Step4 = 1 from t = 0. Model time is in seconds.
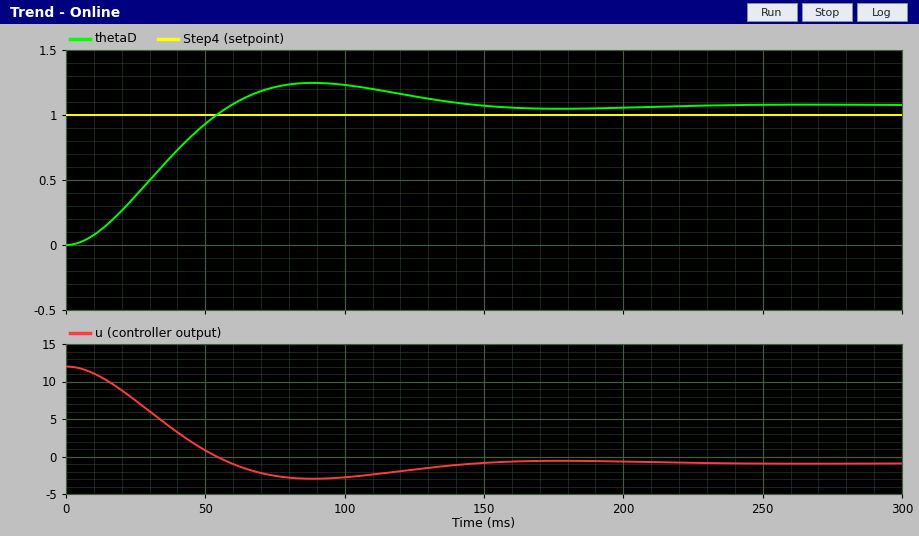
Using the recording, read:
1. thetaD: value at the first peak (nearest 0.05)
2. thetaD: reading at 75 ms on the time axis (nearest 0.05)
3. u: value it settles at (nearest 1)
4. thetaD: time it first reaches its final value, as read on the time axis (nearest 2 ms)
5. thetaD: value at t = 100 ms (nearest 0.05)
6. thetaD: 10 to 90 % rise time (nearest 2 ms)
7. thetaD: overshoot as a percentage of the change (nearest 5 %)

1.25
1.20
-1
60 ms
1.25
40 ms
15 %
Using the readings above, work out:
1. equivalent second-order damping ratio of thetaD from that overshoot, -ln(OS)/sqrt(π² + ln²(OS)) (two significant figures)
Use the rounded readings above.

0.52
